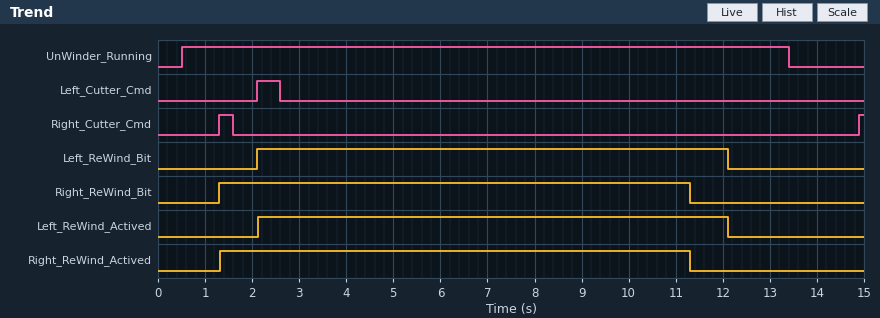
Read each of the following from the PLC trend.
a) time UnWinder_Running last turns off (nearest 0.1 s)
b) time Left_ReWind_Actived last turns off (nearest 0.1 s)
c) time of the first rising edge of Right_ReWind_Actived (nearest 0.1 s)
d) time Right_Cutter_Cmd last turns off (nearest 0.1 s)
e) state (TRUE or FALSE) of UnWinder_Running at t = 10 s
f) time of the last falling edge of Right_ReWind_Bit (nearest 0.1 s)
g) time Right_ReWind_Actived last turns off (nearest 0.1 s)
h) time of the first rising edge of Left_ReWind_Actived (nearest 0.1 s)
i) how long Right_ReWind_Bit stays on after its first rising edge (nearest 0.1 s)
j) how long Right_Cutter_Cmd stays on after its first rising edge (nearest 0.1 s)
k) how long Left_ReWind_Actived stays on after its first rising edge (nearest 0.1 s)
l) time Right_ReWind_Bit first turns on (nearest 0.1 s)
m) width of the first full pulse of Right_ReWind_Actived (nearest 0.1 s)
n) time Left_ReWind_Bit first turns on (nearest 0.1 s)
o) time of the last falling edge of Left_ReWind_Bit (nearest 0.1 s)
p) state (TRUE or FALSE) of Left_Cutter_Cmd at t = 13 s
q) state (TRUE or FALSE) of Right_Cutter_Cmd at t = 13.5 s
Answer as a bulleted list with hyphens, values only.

- 13.4 s
- 12.1 s
- 1.3 s
- 1.6 s
- TRUE
- 11.3 s
- 11.3 s
- 2.1 s
- 10.0 s
- 0.3 s
- 10.0 s
- 1.3 s
- 10.0 s
- 2.1 s
- 12.1 s
- FALSE
- FALSE
